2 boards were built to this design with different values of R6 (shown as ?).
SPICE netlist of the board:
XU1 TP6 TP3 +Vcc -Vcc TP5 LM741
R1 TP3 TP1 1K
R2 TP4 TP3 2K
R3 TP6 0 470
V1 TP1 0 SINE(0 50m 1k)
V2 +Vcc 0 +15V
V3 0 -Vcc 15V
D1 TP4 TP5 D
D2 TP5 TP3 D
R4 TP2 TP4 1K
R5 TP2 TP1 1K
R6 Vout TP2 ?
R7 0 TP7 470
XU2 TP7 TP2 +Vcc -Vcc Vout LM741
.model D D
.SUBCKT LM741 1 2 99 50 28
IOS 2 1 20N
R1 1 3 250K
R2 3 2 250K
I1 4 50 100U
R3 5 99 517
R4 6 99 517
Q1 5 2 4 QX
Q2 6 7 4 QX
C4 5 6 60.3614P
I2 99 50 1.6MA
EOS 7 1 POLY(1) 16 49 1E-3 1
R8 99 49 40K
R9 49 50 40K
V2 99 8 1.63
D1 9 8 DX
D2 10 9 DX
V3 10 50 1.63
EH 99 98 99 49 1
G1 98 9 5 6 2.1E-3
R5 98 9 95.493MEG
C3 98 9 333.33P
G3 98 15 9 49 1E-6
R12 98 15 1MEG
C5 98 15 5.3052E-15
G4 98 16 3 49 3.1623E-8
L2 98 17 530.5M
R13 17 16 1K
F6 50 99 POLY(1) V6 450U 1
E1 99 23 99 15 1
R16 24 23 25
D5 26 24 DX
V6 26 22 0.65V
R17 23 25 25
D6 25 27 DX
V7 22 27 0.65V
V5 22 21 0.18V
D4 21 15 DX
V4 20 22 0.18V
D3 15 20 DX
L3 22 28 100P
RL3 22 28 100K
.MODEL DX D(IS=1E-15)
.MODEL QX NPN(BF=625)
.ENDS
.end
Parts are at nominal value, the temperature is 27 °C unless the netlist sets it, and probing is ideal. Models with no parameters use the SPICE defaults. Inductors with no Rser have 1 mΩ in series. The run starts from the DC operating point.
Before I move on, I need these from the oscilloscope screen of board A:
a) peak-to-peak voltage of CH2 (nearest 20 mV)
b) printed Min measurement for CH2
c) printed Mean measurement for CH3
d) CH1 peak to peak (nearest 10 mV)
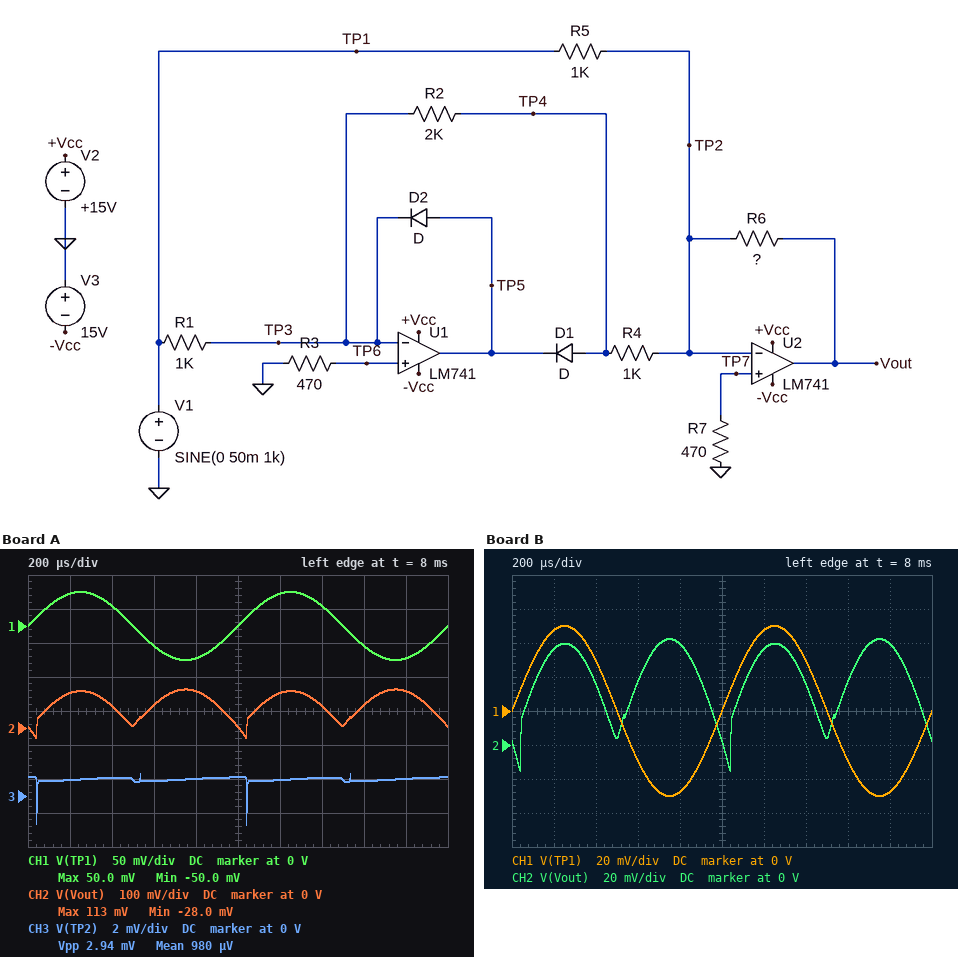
140 mV
-28.0 mV
980 µV
100 mV
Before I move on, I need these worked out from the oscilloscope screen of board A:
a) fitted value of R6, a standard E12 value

2.2 kΩ
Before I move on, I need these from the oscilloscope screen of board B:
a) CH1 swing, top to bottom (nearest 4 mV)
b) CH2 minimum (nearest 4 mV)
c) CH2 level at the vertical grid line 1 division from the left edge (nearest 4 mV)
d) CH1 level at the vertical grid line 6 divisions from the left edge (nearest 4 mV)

100 mV
-16 mV
56 mV
48 mV
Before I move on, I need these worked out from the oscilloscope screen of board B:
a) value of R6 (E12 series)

1.2 kΩ
